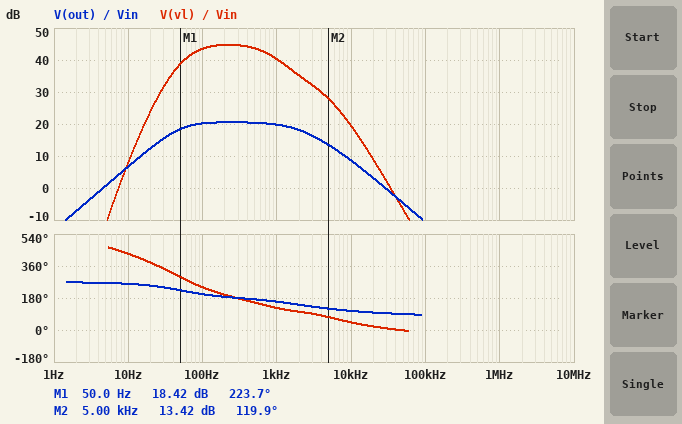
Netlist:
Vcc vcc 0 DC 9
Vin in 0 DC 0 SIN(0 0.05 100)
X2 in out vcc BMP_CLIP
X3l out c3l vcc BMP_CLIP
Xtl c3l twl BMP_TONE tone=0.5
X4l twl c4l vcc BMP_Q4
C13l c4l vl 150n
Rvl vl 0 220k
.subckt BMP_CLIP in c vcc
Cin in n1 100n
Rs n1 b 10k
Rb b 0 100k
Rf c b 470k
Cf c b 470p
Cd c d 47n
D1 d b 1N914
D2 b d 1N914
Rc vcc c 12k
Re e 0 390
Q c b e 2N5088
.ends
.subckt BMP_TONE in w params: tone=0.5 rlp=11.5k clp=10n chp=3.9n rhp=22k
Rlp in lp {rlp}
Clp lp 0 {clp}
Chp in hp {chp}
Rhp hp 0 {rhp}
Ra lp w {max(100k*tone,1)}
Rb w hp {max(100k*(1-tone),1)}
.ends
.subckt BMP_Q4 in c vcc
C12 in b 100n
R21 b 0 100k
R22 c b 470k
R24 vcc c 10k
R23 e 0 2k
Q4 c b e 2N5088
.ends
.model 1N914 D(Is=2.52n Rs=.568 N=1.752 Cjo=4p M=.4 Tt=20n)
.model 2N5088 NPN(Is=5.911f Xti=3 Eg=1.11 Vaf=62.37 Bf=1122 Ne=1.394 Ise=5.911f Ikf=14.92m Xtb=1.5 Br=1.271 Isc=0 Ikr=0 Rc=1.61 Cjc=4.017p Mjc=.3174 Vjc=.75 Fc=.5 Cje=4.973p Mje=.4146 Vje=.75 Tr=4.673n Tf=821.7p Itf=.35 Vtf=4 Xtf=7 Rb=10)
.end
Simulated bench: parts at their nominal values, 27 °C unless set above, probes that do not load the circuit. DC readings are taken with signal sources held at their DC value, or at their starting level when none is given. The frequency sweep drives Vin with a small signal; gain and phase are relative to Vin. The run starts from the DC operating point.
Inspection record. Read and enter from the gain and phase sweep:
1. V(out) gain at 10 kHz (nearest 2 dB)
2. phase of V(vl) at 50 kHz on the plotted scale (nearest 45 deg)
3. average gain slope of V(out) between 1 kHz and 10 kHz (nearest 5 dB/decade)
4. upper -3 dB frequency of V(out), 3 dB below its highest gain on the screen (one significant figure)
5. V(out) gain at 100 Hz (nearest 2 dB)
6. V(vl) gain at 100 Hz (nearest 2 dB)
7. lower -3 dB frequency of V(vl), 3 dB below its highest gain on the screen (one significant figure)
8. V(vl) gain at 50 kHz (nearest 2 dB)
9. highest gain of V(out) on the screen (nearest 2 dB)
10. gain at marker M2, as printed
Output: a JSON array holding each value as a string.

["8 dB", "0 deg", "-10 dB/decade", "2 kHz", "20 dB", "44 dB", "70 Hz", "-6 dB", "20 dB", "13.42 dB"]
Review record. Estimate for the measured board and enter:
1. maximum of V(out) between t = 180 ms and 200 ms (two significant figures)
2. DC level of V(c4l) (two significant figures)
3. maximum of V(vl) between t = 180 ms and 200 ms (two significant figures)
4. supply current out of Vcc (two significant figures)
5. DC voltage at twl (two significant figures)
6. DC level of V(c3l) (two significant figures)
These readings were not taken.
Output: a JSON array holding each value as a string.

["5.0 V", "6.5 V", "850 mV", "970 µA", "2.5 V", "4.6 V"]
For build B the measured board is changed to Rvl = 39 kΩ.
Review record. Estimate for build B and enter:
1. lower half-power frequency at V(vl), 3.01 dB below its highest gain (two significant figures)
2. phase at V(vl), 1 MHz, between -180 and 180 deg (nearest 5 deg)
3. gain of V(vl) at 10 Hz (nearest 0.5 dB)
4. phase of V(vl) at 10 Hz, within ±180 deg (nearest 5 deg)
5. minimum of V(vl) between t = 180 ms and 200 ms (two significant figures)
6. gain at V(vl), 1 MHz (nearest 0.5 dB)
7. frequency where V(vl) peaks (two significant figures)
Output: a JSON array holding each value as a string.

["74 Hz", "-160 deg", "-0.5 dB", "110 deg", "-710 mV", "-54.0 dB", "230 Hz"]
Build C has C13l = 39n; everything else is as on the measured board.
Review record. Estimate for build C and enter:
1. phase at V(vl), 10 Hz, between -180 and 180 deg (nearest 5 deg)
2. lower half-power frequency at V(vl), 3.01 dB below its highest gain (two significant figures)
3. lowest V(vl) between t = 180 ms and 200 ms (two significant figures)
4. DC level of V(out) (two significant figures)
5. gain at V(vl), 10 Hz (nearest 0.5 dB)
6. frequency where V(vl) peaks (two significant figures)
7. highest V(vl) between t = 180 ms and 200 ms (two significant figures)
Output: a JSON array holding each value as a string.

["105 deg", "73 Hz", "-830 mV", "4.7 V", "2.5 dB", "230 Hz", "830 mV"]
